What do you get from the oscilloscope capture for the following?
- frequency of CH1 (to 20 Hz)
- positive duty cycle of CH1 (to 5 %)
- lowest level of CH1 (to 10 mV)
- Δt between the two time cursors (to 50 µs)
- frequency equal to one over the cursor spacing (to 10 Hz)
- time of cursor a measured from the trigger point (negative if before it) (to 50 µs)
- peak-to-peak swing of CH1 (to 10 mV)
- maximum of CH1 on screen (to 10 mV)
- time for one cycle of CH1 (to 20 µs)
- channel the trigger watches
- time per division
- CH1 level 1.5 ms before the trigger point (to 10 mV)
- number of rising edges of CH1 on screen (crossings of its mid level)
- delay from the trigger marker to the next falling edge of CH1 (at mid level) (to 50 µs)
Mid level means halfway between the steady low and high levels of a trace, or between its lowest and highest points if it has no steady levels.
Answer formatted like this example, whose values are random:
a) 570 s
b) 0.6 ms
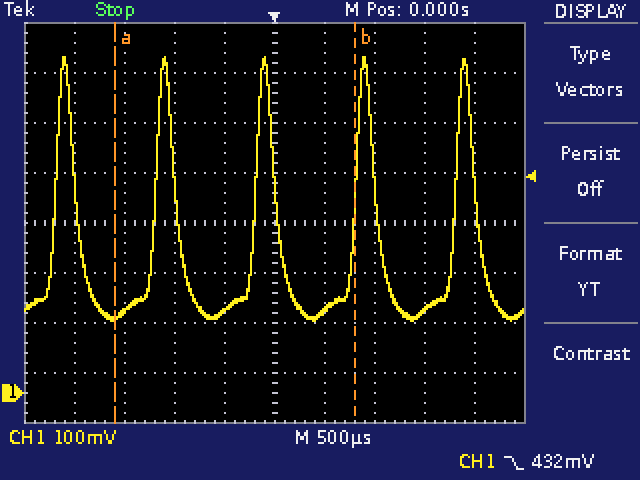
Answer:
a) 1.00 kHz
b) 20 %
c) 140 mV
d) 2.40 ms
e) 420 Hz
f) -1.60 ms
g) 530 mV
h) 670 mV
i) 1.00 ms
j) CH1
k) 500 µs
l) 160 mV
m) 5
n) 1.00 ms
